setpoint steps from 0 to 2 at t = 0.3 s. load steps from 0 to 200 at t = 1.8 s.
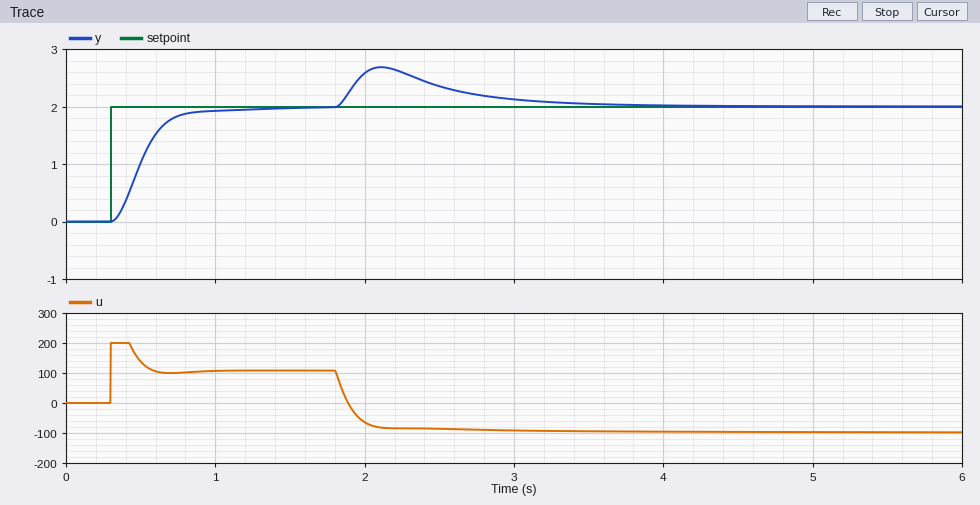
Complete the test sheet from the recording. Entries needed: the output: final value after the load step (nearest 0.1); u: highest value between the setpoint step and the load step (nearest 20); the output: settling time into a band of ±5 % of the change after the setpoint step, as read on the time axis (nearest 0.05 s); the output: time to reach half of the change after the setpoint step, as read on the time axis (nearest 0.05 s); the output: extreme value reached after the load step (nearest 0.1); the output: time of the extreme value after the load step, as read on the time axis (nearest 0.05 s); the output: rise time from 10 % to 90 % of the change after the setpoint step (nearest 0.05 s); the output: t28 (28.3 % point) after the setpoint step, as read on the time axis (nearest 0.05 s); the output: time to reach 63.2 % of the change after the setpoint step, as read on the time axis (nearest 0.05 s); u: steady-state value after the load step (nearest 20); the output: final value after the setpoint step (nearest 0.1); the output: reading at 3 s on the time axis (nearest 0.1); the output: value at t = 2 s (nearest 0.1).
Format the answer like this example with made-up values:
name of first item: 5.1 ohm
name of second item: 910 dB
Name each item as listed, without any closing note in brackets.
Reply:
the output: final value after the load step: 2.0
u: highest value between the setpoint step and the load step: 200
the output: settling time into a band of ±5 % of the change after the setpoint step, as read on the time axis: 0.85 s
the output: time to reach half of the change after the setpoint step, as read on the time axis: 0.50 s
the output: extreme value reached after the load step: 2.7
the output: time of the extreme value after the load step, as read on the time axis: 2.10 s
the output: rise time from 10 % to 90 % of the change after the setpoint step: 0.35 s
the output: t28 (28.3 % point) after the setpoint step, as read on the time axis: 0.45 s
the output: time to reach 63.2 % of the change after the setpoint step, as read on the time axis: 0.55 s
u: steady-state value after the load step: -100
the output: final value after the setpoint step: 2.0
the output: reading at 3 s on the time axis: 2.1
the output: value at t = 2 s: 2.6
